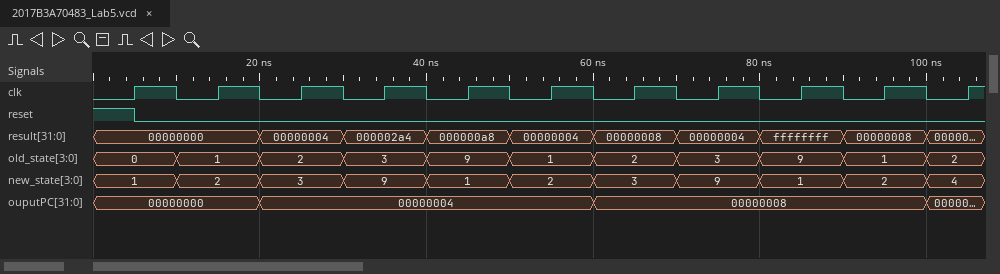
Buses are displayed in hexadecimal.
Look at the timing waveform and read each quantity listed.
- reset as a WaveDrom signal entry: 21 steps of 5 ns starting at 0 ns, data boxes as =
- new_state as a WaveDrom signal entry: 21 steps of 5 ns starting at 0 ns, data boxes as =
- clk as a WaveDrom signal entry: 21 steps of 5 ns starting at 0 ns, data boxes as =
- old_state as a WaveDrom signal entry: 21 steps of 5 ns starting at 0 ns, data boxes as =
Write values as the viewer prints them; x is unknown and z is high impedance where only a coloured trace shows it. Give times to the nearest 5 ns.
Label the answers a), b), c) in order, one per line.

a) {name: 'reset', wave: '10...................'}
b) {name: 'new_state', wave: '=.=.=.=.=.=.=.=.=.=.=', data: '1 2 3 9 1 2 3 9 1 2 4'}
c) {name: 'clk', wave: '010101010101010101010'}
d) {name: 'old_state', wave: '=.=.=.=.=.=.=.=.=.=.=', data: '0 1 2 3 9 1 2 3 9 1 2'}
